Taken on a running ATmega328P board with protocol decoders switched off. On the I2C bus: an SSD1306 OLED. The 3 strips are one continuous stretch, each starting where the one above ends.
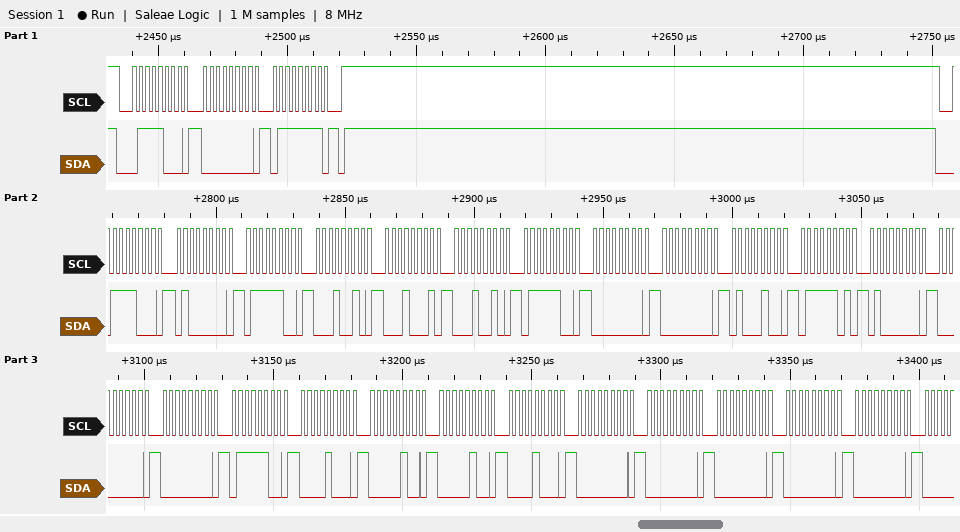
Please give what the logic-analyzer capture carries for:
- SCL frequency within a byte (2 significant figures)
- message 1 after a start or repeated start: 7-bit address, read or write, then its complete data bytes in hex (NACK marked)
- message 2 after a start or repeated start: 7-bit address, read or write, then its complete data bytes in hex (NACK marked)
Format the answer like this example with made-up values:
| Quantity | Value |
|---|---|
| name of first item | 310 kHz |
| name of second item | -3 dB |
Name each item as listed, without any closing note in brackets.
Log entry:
| Quantity | Value |
|---|---|
| SCL frequency within a byte | 400 kHz |
| message 1 after a start or repeated start: 7-bit address, read or write, then its complete data bytes in hex | 0x3C write: 00 7F |
| message 2 after a start or repeated start: 7-bit address, read or write, then its complete data bytes in hex | 0x3C write: 40 7C 12 11 12 7C 00 00 44 7D 40 00 00 7C 08 04 04 08 00 00 00 00 00 |
